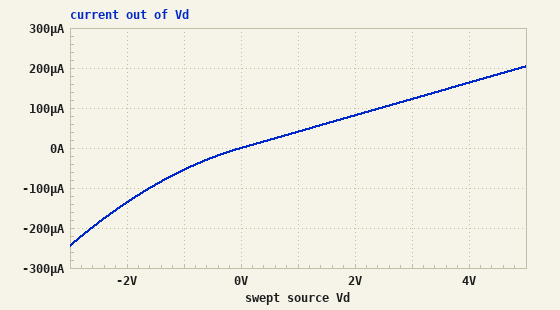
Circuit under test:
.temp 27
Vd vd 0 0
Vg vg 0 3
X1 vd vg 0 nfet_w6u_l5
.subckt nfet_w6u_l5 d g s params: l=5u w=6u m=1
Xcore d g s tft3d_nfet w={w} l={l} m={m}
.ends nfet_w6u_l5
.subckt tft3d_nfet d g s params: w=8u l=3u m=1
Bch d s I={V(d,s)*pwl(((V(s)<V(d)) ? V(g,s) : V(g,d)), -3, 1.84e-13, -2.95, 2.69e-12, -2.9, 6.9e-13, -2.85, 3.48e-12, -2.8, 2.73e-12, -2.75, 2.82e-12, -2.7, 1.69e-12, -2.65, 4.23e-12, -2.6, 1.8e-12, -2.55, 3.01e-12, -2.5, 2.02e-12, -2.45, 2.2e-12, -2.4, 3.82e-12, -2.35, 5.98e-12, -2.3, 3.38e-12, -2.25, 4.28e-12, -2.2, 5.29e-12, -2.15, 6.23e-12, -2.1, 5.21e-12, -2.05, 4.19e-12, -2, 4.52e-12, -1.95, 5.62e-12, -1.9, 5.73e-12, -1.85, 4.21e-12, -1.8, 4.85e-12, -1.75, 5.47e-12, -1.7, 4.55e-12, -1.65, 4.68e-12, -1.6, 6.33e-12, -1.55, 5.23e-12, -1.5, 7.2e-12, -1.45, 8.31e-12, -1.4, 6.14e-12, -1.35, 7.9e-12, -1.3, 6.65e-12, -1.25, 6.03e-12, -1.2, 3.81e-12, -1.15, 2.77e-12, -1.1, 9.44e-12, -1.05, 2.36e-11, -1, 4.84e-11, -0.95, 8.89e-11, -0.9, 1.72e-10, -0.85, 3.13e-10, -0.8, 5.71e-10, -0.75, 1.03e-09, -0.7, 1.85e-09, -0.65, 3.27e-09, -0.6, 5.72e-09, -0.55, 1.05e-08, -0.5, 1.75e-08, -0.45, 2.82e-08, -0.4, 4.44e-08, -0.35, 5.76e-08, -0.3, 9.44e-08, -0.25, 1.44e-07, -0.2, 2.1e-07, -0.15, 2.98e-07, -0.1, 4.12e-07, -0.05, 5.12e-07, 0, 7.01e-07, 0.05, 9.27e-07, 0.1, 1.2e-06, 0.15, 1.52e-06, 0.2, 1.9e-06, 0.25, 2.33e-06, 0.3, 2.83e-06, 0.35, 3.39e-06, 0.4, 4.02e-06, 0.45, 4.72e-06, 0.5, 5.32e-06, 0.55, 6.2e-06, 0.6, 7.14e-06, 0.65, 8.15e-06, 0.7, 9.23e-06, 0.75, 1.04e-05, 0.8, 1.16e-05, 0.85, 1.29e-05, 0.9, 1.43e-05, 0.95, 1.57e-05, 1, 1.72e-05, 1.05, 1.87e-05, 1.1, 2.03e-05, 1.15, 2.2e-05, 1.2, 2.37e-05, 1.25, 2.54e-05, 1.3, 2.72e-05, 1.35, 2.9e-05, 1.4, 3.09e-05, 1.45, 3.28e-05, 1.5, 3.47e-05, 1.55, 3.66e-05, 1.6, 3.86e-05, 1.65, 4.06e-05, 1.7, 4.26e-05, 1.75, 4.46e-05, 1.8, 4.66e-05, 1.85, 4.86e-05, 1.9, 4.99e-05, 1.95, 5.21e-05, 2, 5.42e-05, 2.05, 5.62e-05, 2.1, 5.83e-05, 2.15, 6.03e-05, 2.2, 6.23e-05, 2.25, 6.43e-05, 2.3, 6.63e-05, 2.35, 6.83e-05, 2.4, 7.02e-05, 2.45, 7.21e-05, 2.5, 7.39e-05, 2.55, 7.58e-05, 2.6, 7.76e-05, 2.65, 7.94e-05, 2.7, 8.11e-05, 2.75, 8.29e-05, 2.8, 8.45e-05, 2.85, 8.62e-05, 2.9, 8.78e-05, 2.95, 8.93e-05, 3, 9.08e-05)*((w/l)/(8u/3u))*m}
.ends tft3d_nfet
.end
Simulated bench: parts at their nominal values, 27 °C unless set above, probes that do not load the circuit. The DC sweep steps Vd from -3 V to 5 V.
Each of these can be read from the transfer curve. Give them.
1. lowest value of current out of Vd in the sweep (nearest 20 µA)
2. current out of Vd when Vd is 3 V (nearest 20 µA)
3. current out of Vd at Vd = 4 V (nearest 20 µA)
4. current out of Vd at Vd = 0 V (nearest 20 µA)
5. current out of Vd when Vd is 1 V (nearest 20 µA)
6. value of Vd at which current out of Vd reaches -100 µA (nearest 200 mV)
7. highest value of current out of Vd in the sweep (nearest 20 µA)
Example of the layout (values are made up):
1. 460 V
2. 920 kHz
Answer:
1. -240 µA
2. 120 µA
3. 160 µA
4. 0 A
5. 40 µA
6. -1.6 V
7. 200 µA
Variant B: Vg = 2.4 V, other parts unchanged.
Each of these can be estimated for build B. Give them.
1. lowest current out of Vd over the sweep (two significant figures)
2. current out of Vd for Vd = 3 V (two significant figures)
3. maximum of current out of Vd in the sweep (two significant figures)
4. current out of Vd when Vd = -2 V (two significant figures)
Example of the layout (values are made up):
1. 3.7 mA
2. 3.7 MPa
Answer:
1. -220 µA
2. 95 µA
3. 160 µA
4. -120 µA
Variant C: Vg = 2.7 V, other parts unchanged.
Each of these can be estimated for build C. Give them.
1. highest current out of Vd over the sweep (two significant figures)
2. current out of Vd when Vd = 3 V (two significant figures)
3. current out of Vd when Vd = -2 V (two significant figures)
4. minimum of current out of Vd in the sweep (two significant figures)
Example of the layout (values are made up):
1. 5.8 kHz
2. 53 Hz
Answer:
1. 180 µA
2. 110 µA
3. -130 µA
4. -230 µA
